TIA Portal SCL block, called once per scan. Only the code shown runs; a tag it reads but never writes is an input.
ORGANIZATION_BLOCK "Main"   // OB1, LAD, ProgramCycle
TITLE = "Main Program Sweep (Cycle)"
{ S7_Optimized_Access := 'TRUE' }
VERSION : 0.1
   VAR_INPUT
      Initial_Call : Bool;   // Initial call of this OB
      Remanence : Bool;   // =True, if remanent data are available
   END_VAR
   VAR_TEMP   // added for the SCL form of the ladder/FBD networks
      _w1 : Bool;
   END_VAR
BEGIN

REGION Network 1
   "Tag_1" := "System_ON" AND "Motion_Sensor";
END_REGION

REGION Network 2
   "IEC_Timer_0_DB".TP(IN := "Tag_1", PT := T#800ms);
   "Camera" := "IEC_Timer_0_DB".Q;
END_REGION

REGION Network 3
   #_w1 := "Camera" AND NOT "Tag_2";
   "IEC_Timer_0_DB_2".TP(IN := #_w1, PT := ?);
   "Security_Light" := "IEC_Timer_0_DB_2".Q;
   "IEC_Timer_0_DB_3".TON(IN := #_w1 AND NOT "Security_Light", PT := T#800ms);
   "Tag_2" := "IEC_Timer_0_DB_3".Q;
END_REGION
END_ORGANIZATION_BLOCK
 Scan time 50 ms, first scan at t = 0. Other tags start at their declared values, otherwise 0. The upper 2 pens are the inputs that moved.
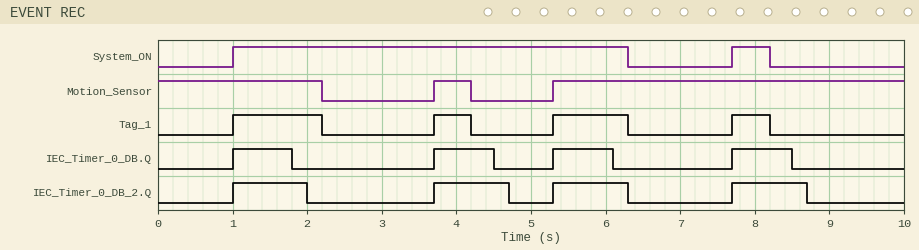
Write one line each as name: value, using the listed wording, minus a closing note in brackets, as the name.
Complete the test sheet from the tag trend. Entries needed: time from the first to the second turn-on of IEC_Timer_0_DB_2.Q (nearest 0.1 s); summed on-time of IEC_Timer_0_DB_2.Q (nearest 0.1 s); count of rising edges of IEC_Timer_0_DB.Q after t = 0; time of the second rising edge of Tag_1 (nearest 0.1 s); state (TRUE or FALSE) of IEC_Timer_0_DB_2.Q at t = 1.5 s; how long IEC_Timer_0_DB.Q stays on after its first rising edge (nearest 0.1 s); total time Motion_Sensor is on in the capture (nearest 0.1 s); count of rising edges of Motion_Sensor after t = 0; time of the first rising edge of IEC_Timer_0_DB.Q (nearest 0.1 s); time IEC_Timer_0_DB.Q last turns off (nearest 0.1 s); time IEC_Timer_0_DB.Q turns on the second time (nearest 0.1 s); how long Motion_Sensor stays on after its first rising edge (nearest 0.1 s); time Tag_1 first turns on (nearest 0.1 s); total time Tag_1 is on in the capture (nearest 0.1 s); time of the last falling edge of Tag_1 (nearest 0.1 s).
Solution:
time from the first to the second turn-on of IEC_Timer_0_DB_2.Q: 2.7 s
summed on-time of IEC_Timer_0_DB_2.Q: 4.0 s
count of rising edges of IEC_Timer_0_DB.Q after t = 0: 4
time of the second rising edge of Tag_1: 3.7 s
state (TRUE or FALSE) of IEC_Timer_0_DB_2.Q at t = 1.5 s: TRUE
how long IEC_Timer_0_DB.Q stays on after its first rising edge: 0.8 s
total time Motion_Sensor is on in the capture: 7.4 s
count of rising edges of Motion_Sensor after t = 0: 2
time of the first rising edge of IEC_Timer_0_DB.Q: 1.0 s
time IEC_Timer_0_DB.Q last turns off: 8.5 s
time IEC_Timer_0_DB.Q turns on the second time: 3.7 s
how long Motion_Sensor stays on after its first rising edge: 0.5 s
time Tag_1 first turns on: 1.0 s
total time Tag_1 is on in the capture: 3.2 s
time of the last falling edge of Tag_1: 8.2 s
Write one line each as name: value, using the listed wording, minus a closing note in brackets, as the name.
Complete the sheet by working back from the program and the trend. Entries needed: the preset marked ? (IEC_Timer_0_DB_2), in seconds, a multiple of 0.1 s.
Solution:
the preset marked ? (IEC_Timer_0_DB_2), in seconds, a multiple of 0.1 s: 1.0 s
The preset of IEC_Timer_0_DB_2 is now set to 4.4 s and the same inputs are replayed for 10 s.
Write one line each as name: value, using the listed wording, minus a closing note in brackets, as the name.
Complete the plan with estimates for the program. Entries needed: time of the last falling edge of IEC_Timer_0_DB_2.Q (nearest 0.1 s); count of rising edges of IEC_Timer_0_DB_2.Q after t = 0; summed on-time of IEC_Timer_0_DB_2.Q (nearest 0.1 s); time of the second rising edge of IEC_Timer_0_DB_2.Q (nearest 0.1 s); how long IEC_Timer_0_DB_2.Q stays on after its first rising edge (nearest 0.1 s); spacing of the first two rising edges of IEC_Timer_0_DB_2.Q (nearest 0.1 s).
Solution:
time of the last falling edge of IEC_Timer_0_DB_2.Q: 5.4 s
count of rising edges of IEC_Timer_0_DB_2.Q after t = 0: 2
summed on-time of IEC_Timer_0_DB_2.Q: 6.7 s
time of the second rising edge of IEC_Timer_0_DB_2.Q: 7.7 s
how long IEC_Timer_0_DB_2.Q stays on after its first rising edge: 4.4 s
spacing of the first two rising edges of IEC_Timer_0_DB_2.Q: 6.7 s
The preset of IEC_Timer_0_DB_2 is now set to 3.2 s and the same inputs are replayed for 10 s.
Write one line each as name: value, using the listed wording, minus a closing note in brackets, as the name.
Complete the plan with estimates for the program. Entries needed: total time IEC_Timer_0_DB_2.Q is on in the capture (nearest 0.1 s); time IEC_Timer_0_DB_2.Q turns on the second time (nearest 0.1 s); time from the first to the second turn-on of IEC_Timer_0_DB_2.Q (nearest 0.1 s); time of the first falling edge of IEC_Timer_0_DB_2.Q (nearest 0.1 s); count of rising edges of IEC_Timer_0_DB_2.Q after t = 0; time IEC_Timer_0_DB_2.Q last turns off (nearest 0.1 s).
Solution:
total time IEC_Timer_0_DB_2.Q is on in the capture: 6.4 s
time IEC_Timer_0_DB_2.Q turns on the second time: 5.3 s
time from the first to the second turn-on of IEC_Timer_0_DB_2.Q: 4.3 s
time of the first falling edge of IEC_Timer_0_DB_2.Q: 4.2 s
count of rising edges of IEC_Timer_0_DB_2.Q after t = 0: 2
time IEC_Timer_0_DB_2.Q last turns off: 8.5 s
